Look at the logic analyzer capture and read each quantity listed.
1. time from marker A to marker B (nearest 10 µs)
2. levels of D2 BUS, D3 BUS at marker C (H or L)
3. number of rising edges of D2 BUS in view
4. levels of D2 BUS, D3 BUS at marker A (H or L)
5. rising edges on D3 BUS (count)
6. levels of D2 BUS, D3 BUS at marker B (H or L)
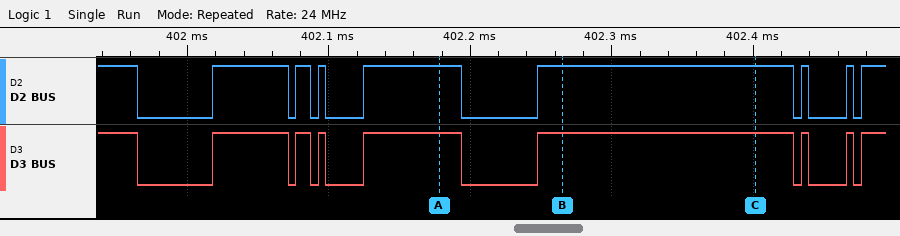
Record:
90 µs
D2 BUS=H, D3 BUS=H
8
D2 BUS=H, D3 BUS=H
8
D2 BUS=H, D3 BUS=H
